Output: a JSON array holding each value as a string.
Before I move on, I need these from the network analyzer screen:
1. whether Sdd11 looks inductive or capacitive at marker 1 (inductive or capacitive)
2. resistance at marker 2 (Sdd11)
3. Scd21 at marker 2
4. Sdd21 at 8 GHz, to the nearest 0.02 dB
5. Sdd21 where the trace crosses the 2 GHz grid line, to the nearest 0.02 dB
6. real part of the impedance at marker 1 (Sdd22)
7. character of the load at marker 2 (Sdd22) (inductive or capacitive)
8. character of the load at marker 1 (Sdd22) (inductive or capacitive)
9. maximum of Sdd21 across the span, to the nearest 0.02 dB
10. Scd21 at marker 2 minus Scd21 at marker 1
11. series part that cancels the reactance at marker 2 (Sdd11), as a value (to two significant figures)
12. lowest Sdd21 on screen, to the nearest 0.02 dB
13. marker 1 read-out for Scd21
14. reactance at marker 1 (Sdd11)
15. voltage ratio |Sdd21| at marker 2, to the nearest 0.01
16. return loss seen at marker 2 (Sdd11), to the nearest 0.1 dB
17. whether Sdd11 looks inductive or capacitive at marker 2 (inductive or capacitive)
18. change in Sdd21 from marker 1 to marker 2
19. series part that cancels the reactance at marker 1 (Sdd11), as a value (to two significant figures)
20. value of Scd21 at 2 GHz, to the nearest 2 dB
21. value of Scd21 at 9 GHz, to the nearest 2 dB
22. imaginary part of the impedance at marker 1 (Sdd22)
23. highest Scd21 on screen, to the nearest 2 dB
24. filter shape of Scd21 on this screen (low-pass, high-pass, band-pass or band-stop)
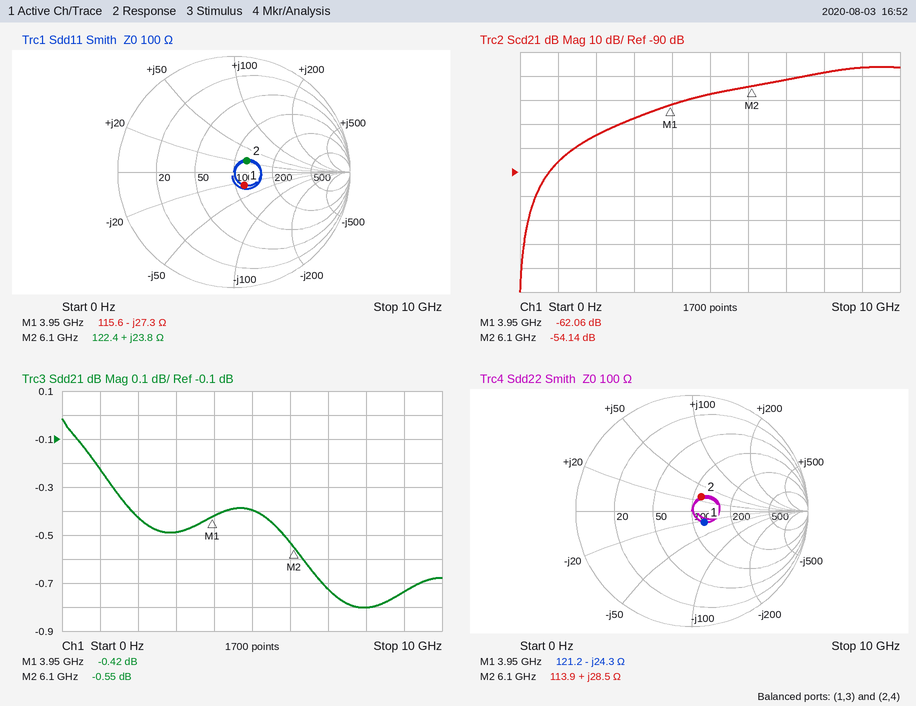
["capacitive", "122.4 Ω", "-54.14 dB", "-0.80 dB", "-0.42 dB", "121.2 Ω", "inductive", "capacitive", "-0.02 dB", "7.92 dB", "1.1 pF", "-0.80 dB", "-62.06 dB", "-27.3 Ω", "0.94", "16.7 dB", "inductive", "-0.13 dB", "1.1 nH", "-74 dB", "-46 dB", "-24.3 Ω", "-46 dB", "high-pass"]
